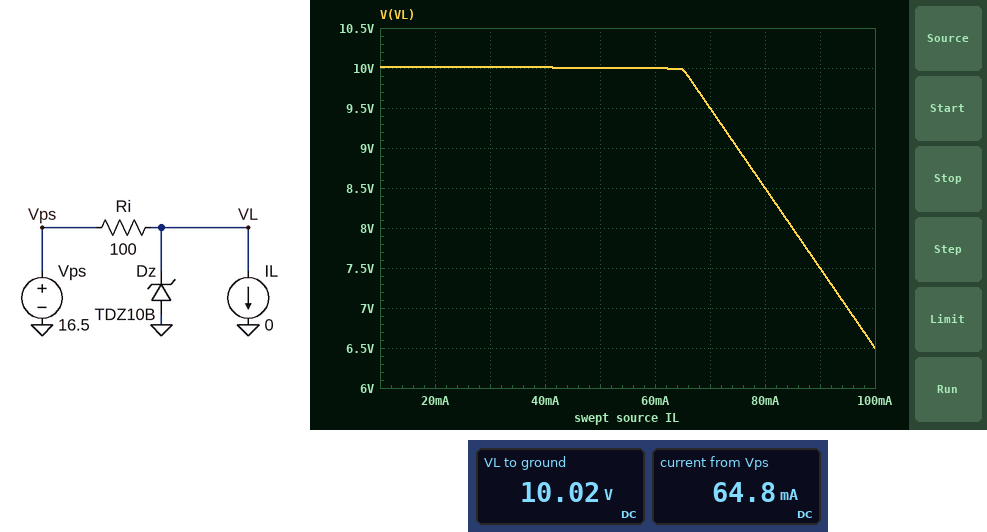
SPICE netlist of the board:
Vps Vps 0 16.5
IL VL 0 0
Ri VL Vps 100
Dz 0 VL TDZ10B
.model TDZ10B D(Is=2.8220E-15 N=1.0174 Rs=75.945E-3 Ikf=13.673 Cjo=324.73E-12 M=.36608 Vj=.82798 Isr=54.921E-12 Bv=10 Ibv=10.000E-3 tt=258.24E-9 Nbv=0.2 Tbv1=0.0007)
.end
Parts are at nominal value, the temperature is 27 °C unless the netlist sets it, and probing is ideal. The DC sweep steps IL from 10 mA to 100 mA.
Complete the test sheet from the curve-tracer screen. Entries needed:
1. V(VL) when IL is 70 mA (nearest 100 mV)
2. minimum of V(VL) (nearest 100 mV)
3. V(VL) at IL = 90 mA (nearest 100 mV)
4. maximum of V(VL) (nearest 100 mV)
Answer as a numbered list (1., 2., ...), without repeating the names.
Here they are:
1. 9.5 V
2. 6.5 V
3. 7.5 V
4. 10.0 V
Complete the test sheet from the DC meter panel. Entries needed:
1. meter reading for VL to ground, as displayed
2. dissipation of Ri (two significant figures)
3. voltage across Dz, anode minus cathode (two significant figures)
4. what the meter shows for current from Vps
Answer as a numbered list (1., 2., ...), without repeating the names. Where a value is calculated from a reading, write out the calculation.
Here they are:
1. 10.02 V
2. (16.5 V - 10.02 V)^2 / 100 Ω = 420 mW
3. 0 V - 10.02 V = -10 V
4. 64.8 mA
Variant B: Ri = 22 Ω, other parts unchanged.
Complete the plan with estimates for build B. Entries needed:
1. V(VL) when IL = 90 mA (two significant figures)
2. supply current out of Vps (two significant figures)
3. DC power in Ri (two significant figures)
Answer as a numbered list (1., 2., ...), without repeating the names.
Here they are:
1. 10 V
2. 290 mA
3. 1.9 W
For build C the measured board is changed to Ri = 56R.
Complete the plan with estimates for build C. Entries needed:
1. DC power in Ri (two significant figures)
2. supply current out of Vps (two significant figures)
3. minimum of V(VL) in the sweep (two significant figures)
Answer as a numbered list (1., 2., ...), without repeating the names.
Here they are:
1. 750 mW
2. 120 mA
3. 10 V
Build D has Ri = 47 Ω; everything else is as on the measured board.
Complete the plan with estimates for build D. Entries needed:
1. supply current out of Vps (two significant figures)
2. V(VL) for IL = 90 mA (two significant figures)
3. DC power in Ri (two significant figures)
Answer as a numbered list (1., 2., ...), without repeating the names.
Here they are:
1. 140 mA
2. 10 V
3. 890 mW
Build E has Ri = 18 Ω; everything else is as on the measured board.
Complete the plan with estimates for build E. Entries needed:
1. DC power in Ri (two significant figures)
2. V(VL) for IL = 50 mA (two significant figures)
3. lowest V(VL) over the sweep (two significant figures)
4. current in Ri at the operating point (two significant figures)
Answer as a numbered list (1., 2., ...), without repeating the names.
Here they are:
1. 2.3 W
2. 10 V
3. 10 V
4. 360 mA
